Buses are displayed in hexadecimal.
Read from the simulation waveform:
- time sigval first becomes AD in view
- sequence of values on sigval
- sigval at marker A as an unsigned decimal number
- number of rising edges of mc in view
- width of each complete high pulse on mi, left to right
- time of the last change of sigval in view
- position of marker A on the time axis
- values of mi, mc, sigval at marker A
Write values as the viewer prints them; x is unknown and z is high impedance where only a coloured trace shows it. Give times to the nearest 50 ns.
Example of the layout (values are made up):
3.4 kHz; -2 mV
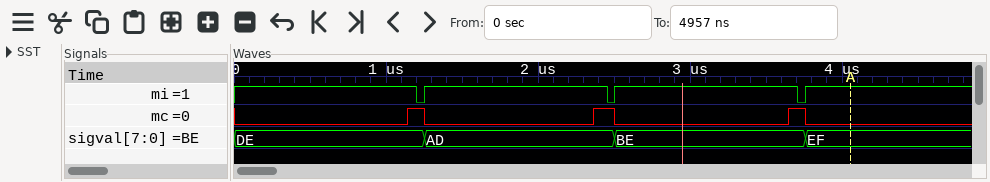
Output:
1250 ns; DE, AD, BE, EF; 239; 3; 1200 ns, 1200 ns; 3750 ns; 4050 ns; mi=1, mc=0, sigval=EF
